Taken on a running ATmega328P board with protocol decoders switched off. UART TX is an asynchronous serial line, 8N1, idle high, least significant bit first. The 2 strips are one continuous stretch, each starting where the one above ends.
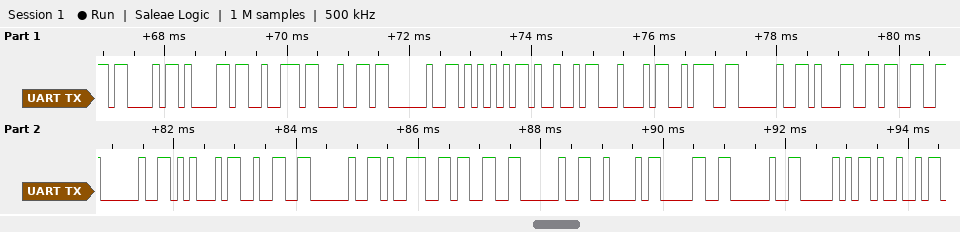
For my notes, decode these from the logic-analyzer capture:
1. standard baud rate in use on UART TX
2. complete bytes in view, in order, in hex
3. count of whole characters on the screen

9600 baud
43 61 72 64 20 55 49 44 3A 20 31 33 20 45 32 20 39 33 20 42 30 20 50 49
24
